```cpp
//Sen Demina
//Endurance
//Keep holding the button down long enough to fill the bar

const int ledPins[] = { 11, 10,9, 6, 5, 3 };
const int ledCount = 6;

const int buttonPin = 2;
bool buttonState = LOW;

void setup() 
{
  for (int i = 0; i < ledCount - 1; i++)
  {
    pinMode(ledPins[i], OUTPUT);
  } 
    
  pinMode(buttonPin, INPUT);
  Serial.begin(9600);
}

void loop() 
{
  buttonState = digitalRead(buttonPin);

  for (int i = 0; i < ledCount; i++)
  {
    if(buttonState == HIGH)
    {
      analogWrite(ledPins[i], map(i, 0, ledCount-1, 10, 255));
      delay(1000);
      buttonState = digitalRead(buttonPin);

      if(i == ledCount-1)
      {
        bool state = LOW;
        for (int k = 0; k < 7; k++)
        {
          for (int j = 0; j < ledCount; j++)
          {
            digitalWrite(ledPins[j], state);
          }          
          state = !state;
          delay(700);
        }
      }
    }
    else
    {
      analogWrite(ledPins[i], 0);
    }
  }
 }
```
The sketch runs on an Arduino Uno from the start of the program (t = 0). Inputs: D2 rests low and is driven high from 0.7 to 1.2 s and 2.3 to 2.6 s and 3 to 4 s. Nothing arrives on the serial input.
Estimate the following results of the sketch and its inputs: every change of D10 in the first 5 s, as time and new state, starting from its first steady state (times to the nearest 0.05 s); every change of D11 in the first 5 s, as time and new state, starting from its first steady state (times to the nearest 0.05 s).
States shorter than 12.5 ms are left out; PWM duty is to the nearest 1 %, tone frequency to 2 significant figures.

0 s low; 3.3 s PWM 23 %; 4.3 s low
0 s low; 0.7 s PWM 4 %; 1.7 s low; 2.3 s PWM 4 %; 4.3 s low
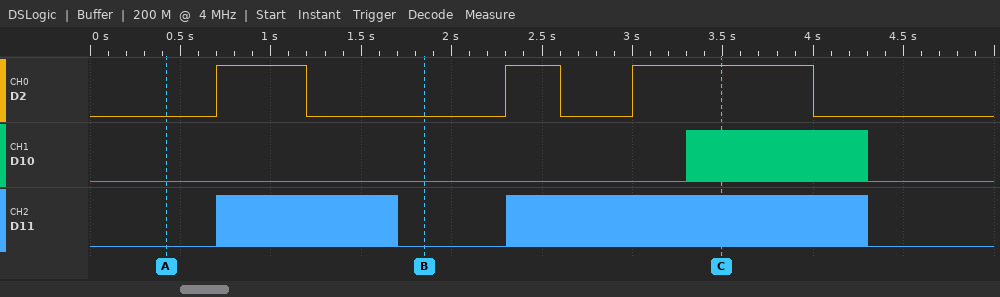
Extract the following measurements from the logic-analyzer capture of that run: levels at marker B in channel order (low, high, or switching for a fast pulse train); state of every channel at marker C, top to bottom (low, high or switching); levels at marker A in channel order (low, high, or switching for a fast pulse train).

D2 low, D10 low, D11 low
D2 high, D10 switching, D11 switching
D2 low, D10 low, D11 low
